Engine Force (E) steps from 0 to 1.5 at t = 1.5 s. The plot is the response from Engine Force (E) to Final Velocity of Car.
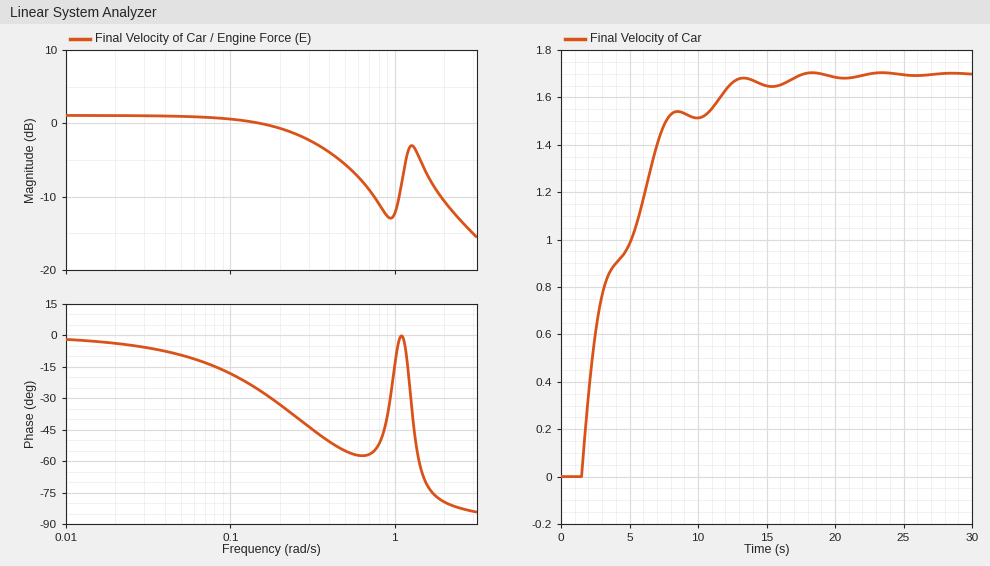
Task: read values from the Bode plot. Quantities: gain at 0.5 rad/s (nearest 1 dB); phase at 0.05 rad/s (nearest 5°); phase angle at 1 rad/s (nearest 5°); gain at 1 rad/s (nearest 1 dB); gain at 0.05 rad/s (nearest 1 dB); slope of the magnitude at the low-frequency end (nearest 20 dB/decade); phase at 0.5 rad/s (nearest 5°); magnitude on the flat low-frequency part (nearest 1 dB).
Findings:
-6 dB
-10°
-15°
-12 dB
1 dB
0 dB/decade
-55°
1 dB
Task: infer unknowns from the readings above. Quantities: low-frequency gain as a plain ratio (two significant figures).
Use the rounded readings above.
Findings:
1.1
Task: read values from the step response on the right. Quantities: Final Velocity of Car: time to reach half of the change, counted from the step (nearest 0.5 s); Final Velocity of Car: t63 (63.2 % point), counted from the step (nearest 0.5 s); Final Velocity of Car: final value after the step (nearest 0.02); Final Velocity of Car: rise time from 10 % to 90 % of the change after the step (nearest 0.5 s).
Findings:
2.0 s
4.0 s
1.70
6.5 s
